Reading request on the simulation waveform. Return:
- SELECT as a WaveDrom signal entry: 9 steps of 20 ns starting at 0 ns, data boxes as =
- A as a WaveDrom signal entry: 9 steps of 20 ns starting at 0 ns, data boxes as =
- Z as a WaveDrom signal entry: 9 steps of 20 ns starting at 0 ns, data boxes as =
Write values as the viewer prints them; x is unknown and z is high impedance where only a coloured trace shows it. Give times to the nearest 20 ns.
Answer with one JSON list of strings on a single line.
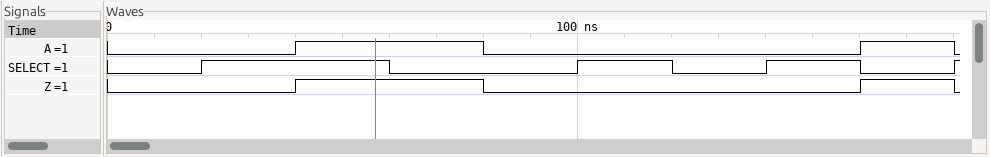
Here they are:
["{name: 'SELECT', wave: '01.0.1010'}", "{name: 'A', wave: '0.1.0...1'}", "{name: 'Z', wave: '0.1.0...1'}"]
